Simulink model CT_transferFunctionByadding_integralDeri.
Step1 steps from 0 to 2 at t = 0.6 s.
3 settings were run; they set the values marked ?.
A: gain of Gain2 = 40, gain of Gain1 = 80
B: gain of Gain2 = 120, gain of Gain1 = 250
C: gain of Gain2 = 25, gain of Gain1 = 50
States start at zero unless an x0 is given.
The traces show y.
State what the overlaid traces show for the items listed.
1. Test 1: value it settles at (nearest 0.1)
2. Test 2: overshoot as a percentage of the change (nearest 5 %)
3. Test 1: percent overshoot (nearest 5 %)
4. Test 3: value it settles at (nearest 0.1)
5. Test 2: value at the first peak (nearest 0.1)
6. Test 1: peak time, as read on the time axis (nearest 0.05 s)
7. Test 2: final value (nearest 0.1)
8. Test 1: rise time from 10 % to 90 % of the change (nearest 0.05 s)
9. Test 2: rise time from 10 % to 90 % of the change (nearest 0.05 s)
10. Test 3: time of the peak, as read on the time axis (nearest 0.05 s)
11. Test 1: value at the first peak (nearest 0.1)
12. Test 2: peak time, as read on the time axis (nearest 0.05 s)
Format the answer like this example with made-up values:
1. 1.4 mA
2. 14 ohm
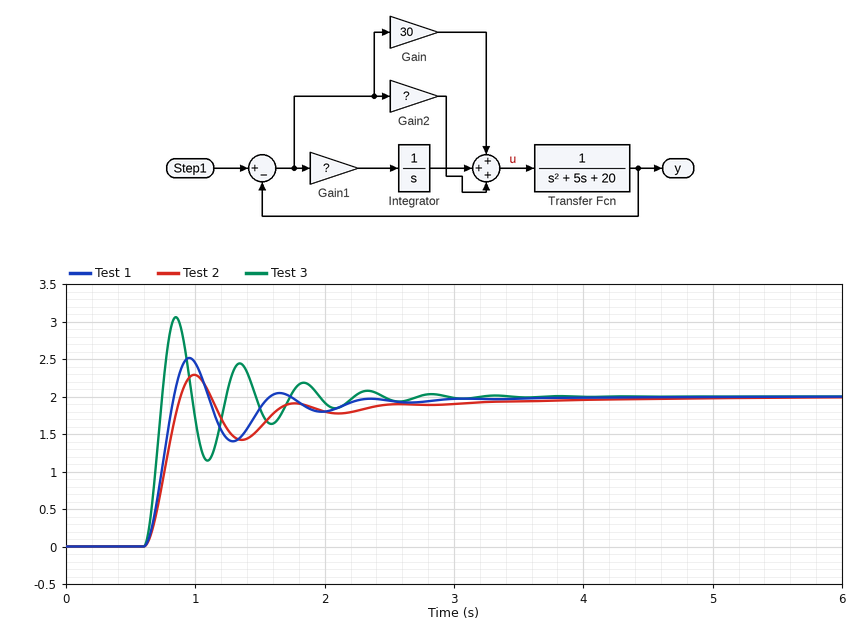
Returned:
1. 2.0
2. 15 %
3. 25 %
4. 2.0
5. 2.3
6. 0.95 s
7. 2.0
8. 0.15 s
9. 0.20 s
10. 0.85 s
11. 2.5
12. 1.00 s
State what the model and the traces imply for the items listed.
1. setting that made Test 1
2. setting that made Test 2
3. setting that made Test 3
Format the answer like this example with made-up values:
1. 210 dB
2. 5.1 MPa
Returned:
1. A
2. C
3. B
